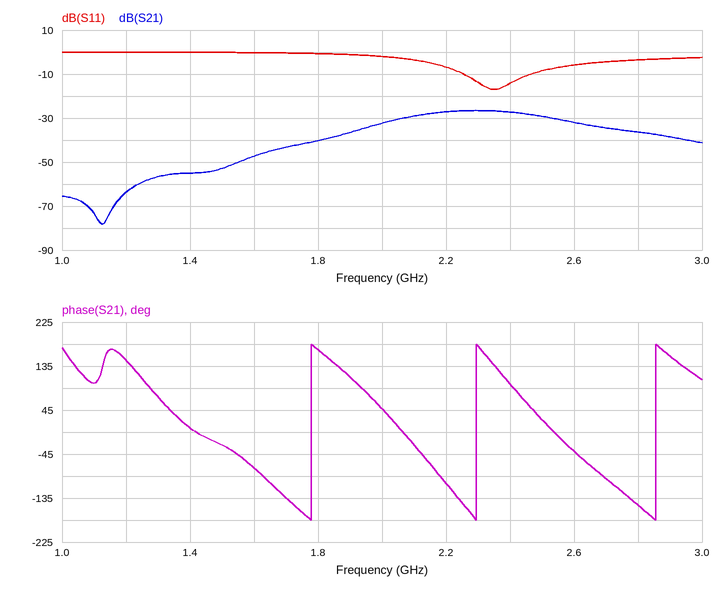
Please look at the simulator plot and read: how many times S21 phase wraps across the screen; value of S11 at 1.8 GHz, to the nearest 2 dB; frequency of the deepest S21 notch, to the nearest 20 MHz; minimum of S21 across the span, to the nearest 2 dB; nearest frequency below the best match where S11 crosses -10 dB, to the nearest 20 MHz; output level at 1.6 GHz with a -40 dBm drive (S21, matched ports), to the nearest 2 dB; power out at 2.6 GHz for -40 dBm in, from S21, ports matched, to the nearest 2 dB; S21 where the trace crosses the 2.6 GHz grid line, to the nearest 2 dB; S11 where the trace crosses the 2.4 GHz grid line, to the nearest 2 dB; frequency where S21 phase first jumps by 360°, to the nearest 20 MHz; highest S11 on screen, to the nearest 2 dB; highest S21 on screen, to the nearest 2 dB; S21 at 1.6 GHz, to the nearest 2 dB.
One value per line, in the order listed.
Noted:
3
0 dB
1.12 GHz
-78 dB
2.26 GHz
-88 dBm
-72 dBm
-32 dB
-14 dB
1.78 GHz
0 dB
-26 dB
-48 dB
